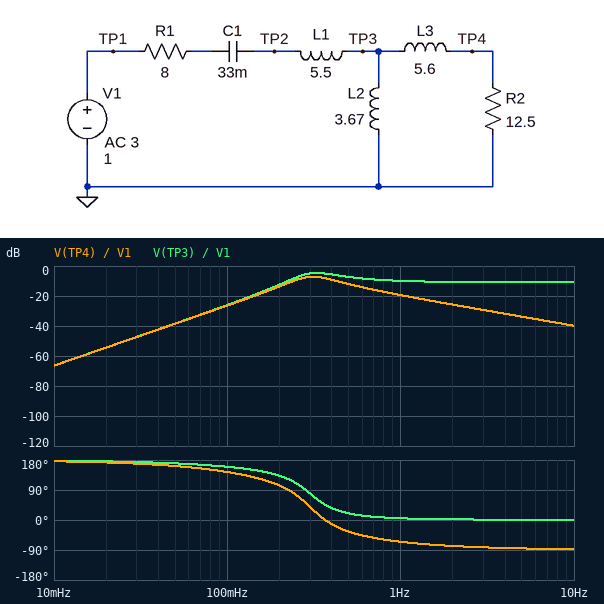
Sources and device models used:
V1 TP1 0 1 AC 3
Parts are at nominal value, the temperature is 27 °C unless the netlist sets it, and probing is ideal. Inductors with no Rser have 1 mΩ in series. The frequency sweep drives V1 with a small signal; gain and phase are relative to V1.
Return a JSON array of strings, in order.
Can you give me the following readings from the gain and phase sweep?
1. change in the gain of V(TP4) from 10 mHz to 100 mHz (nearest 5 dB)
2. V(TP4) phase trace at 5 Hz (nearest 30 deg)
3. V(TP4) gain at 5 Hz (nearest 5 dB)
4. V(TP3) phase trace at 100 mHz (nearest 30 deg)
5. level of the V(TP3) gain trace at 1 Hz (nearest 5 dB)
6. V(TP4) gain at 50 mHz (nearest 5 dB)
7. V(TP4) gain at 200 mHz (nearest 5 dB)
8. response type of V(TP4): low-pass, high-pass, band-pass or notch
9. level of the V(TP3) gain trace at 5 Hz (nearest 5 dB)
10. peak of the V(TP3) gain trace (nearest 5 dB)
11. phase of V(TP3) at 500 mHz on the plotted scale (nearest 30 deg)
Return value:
["40 dB", "-90 deg", "-35 dB", "150 deg", "-10 dB", "-40 dB", "-15 dB", "band-pass", "-10 dB", "-5 dB", "30 deg"]
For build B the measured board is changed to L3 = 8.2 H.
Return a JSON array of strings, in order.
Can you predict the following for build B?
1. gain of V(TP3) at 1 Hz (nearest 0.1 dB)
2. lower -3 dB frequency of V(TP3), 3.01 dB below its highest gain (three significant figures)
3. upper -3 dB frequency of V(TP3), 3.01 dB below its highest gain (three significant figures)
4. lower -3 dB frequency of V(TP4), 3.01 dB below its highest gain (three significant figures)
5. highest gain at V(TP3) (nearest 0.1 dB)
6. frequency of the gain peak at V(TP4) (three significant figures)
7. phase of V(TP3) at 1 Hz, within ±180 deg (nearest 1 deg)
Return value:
["-9.2 dB", "253 mHz", "524 mHz", "237 mHz", "-4.1 dB", "309 mHz", "7 deg"]
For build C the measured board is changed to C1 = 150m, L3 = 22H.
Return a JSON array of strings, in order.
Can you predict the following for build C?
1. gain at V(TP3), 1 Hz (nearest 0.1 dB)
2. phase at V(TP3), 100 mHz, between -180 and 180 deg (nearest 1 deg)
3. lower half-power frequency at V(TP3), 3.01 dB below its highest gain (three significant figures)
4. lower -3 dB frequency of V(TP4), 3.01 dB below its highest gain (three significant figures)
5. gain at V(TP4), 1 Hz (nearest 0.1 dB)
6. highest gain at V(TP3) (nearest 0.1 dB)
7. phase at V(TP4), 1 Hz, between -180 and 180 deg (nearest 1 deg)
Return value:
["-8.7 dB", "117 deg", "118 mHz", "93.9 mHz", "-29.6 dB", "-7.8 dB", "-77 deg"]
